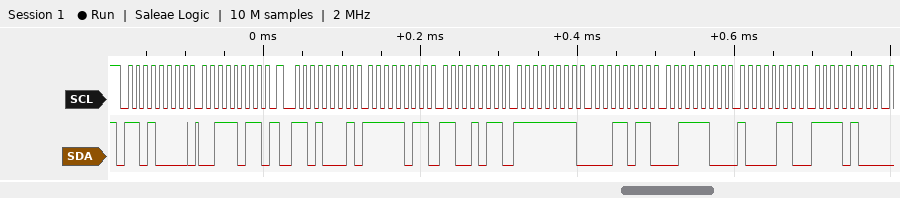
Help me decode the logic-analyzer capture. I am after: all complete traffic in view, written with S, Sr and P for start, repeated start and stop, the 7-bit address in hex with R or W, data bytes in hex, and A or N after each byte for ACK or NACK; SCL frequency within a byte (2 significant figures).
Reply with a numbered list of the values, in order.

1. S 68W A 3B A Sr 68R A FB A CB A FF A 1B A 3C A 86 A F4 A
2. 100 kHz
